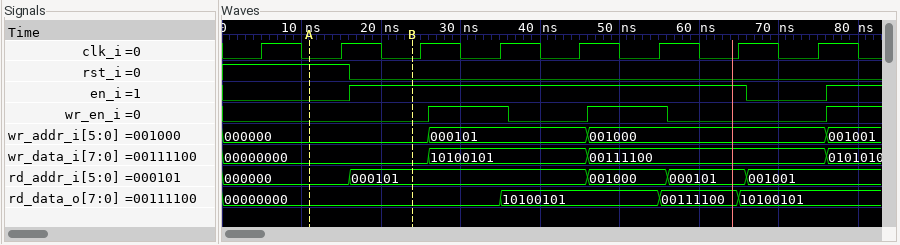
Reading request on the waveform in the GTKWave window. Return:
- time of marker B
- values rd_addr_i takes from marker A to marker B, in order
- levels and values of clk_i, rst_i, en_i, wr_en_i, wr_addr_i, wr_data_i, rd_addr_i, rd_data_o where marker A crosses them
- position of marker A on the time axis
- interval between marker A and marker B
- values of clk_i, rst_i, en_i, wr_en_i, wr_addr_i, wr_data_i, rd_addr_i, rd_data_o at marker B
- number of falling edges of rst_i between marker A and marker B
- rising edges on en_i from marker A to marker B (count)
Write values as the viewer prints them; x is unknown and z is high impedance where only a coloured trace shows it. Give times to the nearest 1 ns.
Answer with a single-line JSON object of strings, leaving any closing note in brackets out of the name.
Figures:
{"time of marker B": "24 ns", "values rd_addr_i takes from marker A to marker B, in order": "000000, 000101", "levels and values of clk_i, rst_i, en_i, wr_en_i, wr_addr_i, wr_data_i, rd_addr_i, rd_data_o where marker A crosses them": "clk_i=0, rst_i=1, en_i=0, wr_en_i=0, wr_addr_i=000000, wr_data_i=00000000, rd_addr_i=000000, rd_data_o=00000000", "position of marker A on the time axis": "11 ns", "interval between marker A and marker B": "13 ns", "values of clk_i, rst_i, en_i, wr_en_i, wr_addr_i, wr_data_i, rd_addr_i, rd_data_o at marker B": "clk_i=0, rst_i=0, en_i=1, wr_en_i=0, wr_addr_i=000000, wr_data_i=00000000, rd_addr_i=000101, rd_data_o=00000000", "number of falling edges of rst_i between marker A and marker B": "1", "rising edges on en_i from marker A to marker B": "1"}
